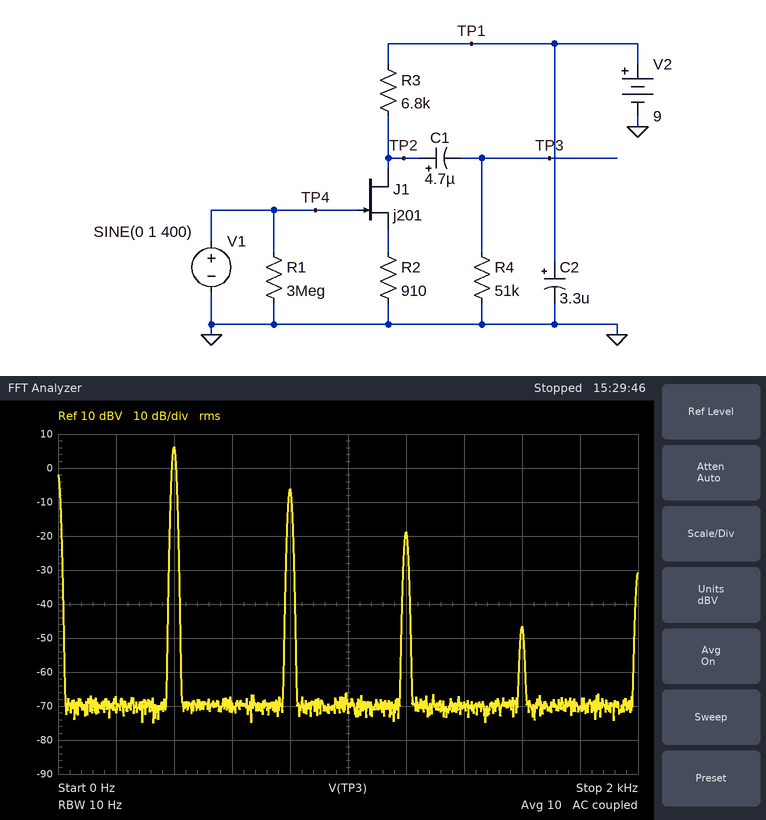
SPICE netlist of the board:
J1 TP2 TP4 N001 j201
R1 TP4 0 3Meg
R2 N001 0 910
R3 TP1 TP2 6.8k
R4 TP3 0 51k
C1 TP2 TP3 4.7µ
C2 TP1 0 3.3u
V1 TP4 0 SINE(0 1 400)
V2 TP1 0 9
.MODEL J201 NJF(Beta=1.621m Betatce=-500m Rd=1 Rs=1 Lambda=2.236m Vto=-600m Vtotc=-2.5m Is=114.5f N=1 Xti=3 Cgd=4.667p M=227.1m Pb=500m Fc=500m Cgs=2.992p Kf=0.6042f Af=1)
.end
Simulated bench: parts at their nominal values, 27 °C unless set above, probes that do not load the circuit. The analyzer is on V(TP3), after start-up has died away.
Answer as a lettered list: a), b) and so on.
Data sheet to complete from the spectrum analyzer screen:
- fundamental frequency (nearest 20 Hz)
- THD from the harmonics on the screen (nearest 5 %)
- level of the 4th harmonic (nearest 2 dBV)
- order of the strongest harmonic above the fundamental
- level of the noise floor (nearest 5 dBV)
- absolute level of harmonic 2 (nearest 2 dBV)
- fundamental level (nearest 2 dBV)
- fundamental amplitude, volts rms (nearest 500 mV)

a) 400 Hz
b) 25 %
c) -46 dBV
d) 2
e) -70 dBV
f) -6 dBV
g) 6 dBV
h) 2.0 V
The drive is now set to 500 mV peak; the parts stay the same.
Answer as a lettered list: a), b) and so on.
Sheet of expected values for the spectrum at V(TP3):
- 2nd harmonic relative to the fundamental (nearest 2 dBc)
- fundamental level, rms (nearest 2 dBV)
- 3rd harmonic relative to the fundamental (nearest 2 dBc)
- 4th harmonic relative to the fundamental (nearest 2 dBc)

a) -22 dBc
b) 2 dBV
c) -36 dBc
d) -48 dBc
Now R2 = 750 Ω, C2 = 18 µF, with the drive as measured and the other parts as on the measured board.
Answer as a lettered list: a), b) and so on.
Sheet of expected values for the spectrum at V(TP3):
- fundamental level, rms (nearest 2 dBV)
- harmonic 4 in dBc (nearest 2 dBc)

a) 8 dBV
b) -48 dBc
